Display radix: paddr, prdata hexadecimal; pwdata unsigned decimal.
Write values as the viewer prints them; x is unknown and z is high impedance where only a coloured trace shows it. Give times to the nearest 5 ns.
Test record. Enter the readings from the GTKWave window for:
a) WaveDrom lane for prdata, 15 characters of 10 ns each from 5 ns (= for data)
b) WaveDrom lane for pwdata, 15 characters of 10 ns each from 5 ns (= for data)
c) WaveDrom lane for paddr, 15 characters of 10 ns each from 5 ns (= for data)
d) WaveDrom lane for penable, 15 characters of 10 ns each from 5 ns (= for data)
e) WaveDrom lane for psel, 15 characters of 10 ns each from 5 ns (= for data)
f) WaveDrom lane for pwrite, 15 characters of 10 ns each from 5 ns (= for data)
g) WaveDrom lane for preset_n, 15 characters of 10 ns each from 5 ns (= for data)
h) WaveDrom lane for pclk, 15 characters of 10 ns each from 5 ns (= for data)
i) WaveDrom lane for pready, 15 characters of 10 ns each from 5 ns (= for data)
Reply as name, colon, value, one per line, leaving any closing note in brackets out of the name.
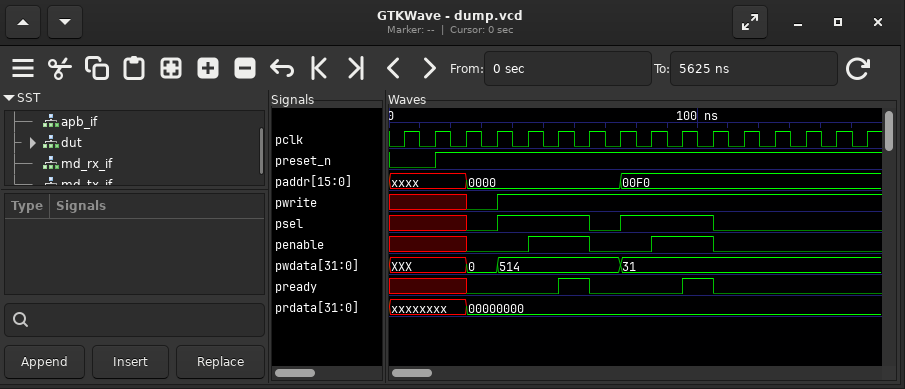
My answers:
WaveDrom lane for prdata, 15 characters of 10 ns each from 5 ns: {name: 'prdata', wave: 'x.=............', data: '00000000'}
WaveDrom lane for pwdata, 15 characters of 10 ns each from 5 ns: {name: 'pwdata', wave: 'x.==...=.......', data: '0 514 31'}
WaveDrom lane for paddr, 15 characters of 10 ns each from 5 ns: {name: 'paddr', wave: 'x.=....=.......', data: '0000 00F0'}
WaveDrom lane for penable, 15 characters of 10 ns each from 5 ns: {name: 'penable', wave: 'x.0.1.0.1.0....'}
WaveDrom lane for psel, 15 characters of 10 ns each from 5 ns: {name: 'psel', wave: 'x.01..01..0....'}
WaveDrom lane for pwrite, 15 characters of 10 ns each from 5 ns: {name: 'pwrite', wave: 'x.01...........'}
WaveDrom lane for preset_n, 15 characters of 10 ns each from 5 ns: {name: 'preset_n', wave: '01.............'}
WaveDrom lane for pclk, 15 characters of 10 ns each from 5 ns: {name: 'pclk', wave: 'p..............'}
WaveDrom lane for pready, 15 characters of 10 ns each from 5 ns: {name: 'pready', wave: 'x.0..10..10....'}
